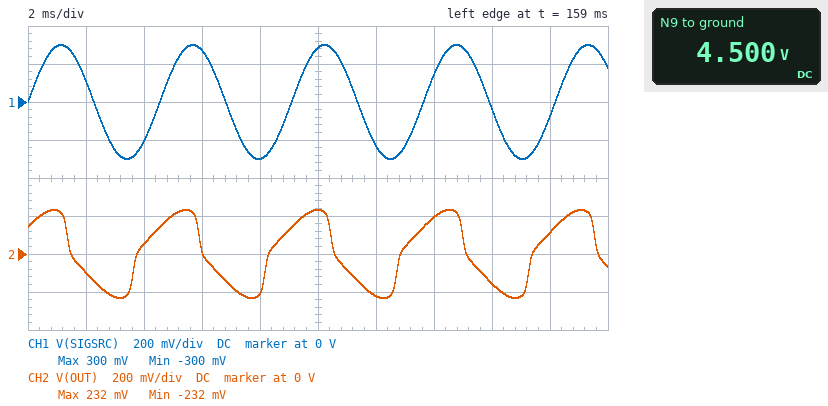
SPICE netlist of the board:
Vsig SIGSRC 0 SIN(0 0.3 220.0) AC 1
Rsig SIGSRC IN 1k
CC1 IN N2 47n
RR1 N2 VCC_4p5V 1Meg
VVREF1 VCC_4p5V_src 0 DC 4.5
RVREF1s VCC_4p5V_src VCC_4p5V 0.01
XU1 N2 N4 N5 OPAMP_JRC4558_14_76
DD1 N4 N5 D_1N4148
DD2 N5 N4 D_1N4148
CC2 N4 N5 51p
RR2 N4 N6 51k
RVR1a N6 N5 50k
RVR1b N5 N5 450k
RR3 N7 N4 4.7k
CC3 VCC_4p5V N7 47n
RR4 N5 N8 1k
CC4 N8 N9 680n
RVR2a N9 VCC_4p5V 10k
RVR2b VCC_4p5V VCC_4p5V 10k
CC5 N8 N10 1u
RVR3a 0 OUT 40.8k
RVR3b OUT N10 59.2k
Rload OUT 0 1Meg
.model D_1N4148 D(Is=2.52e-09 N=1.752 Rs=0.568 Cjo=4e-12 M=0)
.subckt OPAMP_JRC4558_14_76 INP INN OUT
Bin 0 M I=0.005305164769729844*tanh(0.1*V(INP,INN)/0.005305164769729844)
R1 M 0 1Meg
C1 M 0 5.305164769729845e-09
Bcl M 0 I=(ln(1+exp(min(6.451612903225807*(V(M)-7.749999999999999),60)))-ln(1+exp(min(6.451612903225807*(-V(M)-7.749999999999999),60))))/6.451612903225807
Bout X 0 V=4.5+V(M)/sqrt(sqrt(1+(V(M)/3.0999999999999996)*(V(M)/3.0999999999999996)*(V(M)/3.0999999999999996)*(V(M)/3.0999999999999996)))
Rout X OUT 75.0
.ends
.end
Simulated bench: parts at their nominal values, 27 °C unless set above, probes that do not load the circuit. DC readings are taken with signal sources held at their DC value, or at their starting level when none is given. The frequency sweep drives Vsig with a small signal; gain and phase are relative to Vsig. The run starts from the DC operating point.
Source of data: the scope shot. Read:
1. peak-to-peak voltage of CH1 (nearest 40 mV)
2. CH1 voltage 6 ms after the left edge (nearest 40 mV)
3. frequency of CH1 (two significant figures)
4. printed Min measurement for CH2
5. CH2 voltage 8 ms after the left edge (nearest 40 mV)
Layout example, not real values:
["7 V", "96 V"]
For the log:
["600 mV", "280 mV", "220 Hz", "-232 mV", "-200 mV"]
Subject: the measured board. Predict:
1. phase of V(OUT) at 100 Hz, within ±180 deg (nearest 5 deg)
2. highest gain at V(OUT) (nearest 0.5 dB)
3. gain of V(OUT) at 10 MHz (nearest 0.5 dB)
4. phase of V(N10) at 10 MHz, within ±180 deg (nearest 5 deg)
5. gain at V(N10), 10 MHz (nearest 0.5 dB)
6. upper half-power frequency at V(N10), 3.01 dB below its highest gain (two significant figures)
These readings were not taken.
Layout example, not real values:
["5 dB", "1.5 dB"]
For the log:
["65 deg", "18.0 dB", "-20.0 dB", "-75 deg", "-12.0 dB", "24 kHz"]
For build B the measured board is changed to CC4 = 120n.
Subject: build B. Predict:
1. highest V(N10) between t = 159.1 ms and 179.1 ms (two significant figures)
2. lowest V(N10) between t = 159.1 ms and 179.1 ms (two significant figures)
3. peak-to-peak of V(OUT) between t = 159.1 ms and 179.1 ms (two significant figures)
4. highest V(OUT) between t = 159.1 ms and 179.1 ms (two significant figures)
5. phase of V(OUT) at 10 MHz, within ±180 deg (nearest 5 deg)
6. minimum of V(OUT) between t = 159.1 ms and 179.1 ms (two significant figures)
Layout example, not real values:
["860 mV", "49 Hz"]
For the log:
["600 mV", "-600 mV", "480 mV", "240 mV", "-75 deg", "-240 mV"]
